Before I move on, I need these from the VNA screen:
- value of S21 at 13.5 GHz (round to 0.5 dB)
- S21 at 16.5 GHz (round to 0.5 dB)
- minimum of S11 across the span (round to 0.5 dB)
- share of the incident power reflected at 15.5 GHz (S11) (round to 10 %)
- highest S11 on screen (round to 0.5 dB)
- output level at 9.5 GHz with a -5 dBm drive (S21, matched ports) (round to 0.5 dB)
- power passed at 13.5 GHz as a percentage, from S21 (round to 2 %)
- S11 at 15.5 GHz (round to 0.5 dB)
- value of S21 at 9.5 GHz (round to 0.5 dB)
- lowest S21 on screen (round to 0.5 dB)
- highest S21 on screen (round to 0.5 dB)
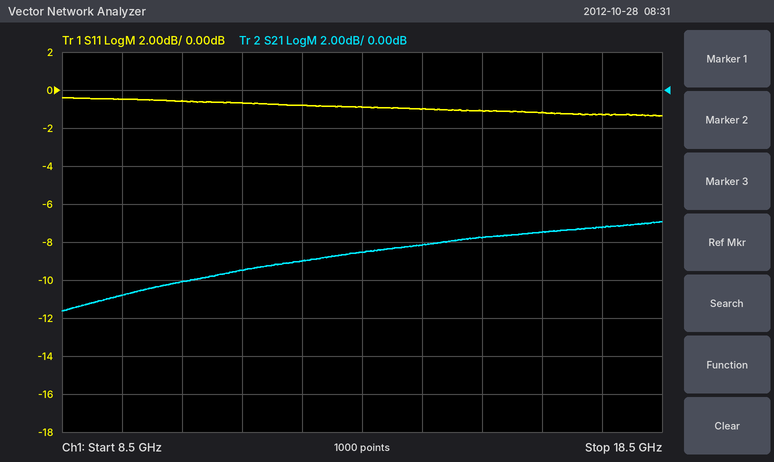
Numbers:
-8.5 dB
-7.5 dB
-1.5 dB
80 %
-0.5 dB
-16.0 dBm
14 %
-1.0 dB
-11.0 dB
-11.5 dB
-7.0 dB
